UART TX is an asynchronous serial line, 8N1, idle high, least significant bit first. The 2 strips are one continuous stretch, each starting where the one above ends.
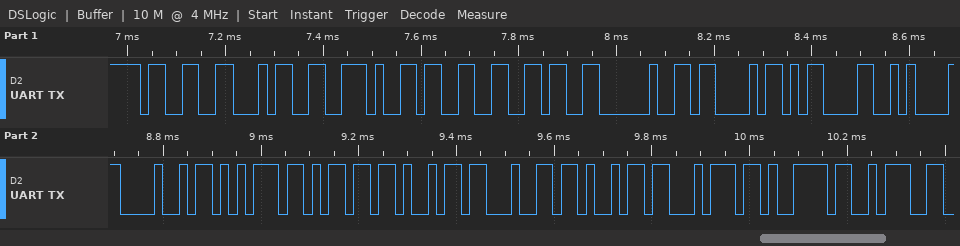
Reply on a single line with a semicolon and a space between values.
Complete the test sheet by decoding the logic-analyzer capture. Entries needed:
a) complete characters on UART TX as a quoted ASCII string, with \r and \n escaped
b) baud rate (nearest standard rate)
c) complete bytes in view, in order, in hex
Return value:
"34.36 C\r\nHumidity:"; 57600 baud; 0x33 0x34 0x2E 0x33 0x36 0x20 0x43 0x0D 0x0A 0x48 0x75 0x6D 0x69 0x64 0x69 0x74 0x79 0x3A
